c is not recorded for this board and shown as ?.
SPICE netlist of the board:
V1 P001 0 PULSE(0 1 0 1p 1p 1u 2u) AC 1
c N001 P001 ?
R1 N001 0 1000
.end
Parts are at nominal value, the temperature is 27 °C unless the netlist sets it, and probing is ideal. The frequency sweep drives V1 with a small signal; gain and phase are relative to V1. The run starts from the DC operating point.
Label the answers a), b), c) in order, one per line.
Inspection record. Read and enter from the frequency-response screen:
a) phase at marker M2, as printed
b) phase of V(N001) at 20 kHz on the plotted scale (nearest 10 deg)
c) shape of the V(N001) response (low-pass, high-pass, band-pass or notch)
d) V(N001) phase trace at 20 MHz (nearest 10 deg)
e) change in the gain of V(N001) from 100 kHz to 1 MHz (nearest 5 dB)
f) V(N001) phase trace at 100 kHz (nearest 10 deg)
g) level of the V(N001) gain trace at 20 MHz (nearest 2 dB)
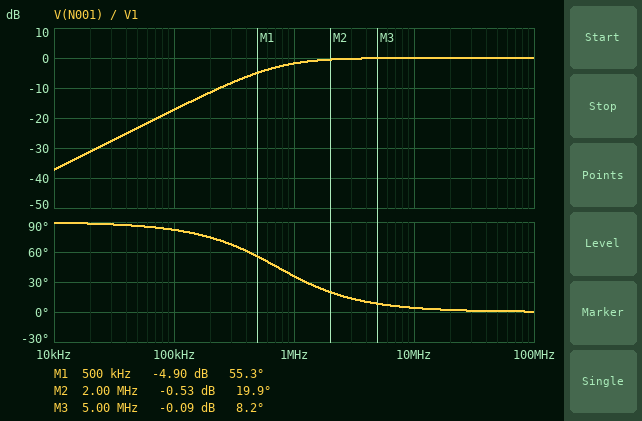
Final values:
a) 19.9 deg
b) 90 deg
c) high-pass
d) 0 deg
e) 15 dB
f) 80 deg
g) 0 dB
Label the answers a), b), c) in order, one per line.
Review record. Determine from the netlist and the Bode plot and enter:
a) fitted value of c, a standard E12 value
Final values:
a) 220 pF
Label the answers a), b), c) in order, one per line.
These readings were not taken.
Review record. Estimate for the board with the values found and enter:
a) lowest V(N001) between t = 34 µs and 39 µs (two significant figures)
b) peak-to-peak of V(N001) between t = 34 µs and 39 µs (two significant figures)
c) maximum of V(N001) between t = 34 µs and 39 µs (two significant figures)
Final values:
a) -990 mV
b) 2.0 V
c) 990 mV
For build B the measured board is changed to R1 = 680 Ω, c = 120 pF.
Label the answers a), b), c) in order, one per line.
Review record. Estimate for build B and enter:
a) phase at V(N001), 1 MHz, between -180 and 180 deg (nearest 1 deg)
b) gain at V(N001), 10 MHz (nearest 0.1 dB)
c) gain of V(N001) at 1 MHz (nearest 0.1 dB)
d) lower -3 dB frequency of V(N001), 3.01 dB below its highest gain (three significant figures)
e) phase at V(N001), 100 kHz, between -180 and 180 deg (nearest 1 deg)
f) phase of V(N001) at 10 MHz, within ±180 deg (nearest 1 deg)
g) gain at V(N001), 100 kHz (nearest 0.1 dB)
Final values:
a) 63 deg
b) -0.2 dB
c) -6.8 dB
d) 1.95 MHz
e) 87 deg
f) 11 deg
g) -25.8 dB
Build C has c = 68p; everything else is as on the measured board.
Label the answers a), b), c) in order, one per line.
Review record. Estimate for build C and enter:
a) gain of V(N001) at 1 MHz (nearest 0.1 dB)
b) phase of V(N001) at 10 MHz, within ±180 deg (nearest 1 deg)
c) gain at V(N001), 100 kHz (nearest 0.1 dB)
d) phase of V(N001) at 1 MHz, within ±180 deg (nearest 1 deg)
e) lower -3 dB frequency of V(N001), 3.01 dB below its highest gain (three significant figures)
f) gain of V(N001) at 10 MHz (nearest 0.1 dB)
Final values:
a) -8.1 dB
b) 13 deg
c) -27.4 dB
d) 67 deg
e) 2.34 MHz
f) -0.2 dB
